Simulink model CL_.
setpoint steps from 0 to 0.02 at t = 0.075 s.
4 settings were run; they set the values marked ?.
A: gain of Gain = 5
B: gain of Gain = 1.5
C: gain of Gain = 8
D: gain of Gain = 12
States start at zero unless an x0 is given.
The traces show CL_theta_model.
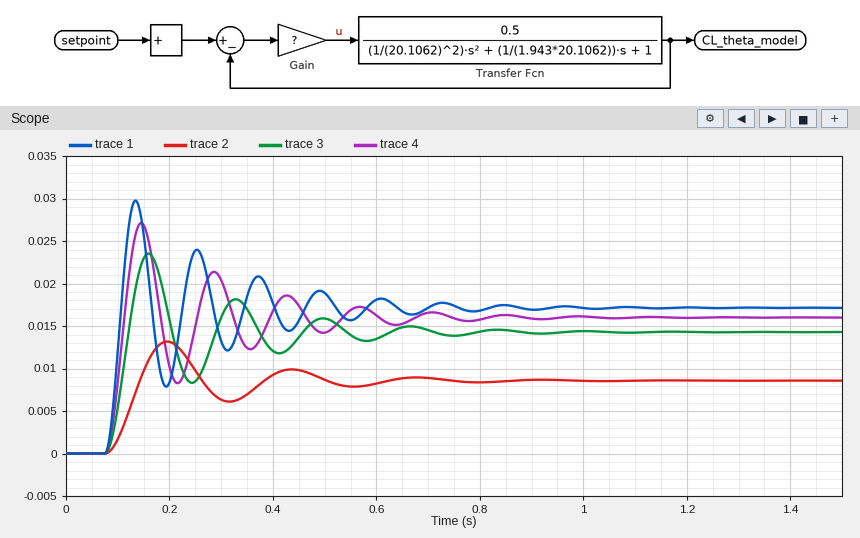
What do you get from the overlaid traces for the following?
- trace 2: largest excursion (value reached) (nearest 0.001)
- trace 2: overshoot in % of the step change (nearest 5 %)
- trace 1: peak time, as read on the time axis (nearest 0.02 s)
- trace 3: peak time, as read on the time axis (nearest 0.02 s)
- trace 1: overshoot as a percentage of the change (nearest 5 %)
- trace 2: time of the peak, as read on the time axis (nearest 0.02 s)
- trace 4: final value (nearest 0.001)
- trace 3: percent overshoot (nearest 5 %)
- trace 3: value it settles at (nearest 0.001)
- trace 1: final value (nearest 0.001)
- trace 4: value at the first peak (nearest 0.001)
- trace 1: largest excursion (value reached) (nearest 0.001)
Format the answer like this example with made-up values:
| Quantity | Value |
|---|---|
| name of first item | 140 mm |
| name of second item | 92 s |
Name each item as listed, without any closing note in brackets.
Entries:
| Quantity | Value |
|---|---|
| trace 2: largest excursion (value reached) | 0.013 |
| trace 2: overshoot in % of the step change | 55 % |
| trace 1: peak time, as read on the time axis | 0.14 s |
| trace 3: peak time, as read on the time axis | 0.16 s |
| trace 1: overshoot as a percentage of the change | 75 % |
| trace 2: time of the peak, as read on the time axis | 0.20 s |
| trace 4: final value | 0.016 |
| trace 3: percent overshoot | 65 % |
| trace 3: value it settles at | 0.014 |
| trace 1: final value | 0.017 |
| trace 4: value at the first peak | 0.027 |
| trace 1: largest excursion (value reached) | 0.030 |
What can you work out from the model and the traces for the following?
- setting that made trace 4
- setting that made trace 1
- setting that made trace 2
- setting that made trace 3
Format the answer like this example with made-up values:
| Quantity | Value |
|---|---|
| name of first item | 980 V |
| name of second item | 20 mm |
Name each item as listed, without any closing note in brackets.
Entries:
| Quantity | Value |
|---|---|
| setting that made trace 4 | C |
| setting that made trace 1 | D |
| setting that made trace 2 | B |
| setting that made trace 3 | A |
